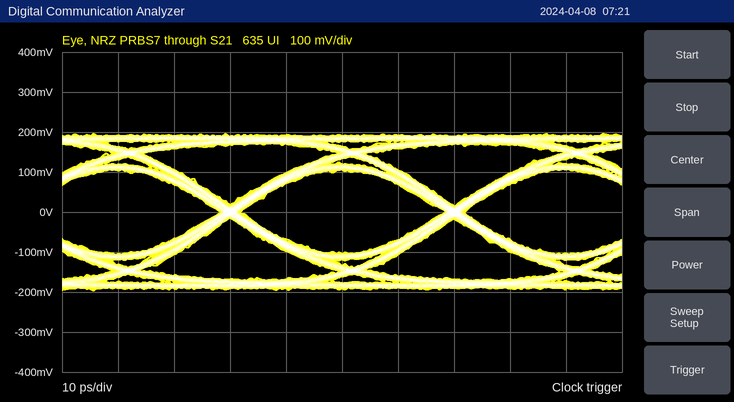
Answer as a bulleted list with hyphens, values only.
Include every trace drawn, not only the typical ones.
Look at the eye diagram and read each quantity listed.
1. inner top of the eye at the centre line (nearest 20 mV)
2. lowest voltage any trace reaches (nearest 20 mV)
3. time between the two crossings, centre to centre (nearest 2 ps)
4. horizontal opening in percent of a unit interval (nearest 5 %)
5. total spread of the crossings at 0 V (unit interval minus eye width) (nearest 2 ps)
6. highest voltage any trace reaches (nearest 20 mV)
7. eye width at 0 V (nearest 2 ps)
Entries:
- 100 mV
- -200 mV
- 40 ps
- 90 %
- 4 ps
- 200 mV
- 36 ps
